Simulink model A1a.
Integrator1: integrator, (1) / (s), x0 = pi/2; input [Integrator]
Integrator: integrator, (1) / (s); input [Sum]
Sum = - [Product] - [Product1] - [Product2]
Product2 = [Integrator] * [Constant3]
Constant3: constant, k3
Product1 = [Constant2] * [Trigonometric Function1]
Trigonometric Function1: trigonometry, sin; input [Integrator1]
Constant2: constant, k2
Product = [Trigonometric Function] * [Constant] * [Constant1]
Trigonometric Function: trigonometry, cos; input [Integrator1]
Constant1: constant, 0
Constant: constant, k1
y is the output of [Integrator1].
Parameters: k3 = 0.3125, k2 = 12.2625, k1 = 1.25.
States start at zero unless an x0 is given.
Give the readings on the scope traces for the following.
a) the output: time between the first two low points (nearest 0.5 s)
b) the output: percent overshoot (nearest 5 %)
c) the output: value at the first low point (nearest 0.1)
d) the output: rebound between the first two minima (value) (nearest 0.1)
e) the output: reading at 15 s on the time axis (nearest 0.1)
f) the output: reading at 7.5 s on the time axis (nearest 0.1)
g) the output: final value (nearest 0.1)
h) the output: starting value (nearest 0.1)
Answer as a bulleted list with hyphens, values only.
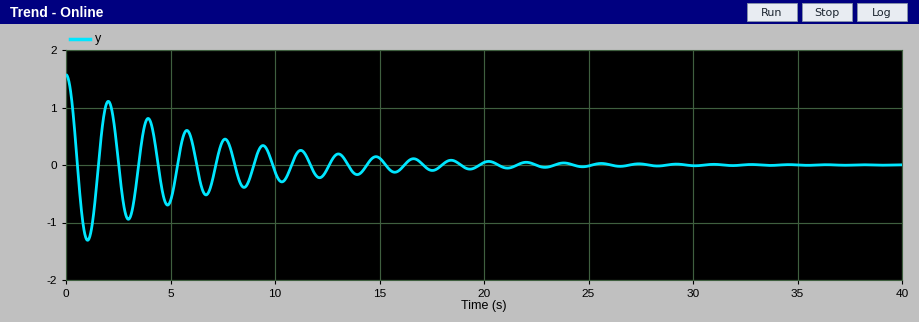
- 2.0 s
- 85 %
- -1.3
- 1.1
- 0.1
- 0.4
- 0.0
- 1.6
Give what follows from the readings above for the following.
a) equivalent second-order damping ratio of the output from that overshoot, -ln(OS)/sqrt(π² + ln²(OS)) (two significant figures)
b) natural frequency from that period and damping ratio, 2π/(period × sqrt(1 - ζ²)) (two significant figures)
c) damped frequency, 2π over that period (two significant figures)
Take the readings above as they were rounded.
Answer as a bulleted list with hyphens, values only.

- 0.052
- 3.1 rad/s
- 3.1 rad/s
